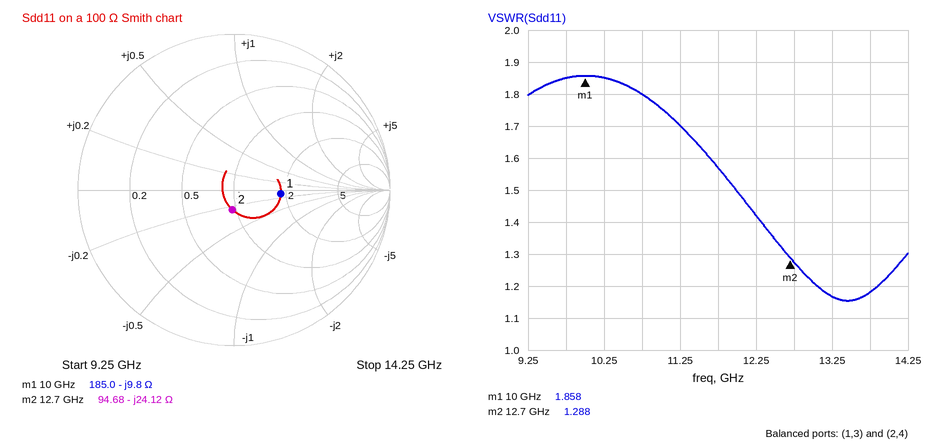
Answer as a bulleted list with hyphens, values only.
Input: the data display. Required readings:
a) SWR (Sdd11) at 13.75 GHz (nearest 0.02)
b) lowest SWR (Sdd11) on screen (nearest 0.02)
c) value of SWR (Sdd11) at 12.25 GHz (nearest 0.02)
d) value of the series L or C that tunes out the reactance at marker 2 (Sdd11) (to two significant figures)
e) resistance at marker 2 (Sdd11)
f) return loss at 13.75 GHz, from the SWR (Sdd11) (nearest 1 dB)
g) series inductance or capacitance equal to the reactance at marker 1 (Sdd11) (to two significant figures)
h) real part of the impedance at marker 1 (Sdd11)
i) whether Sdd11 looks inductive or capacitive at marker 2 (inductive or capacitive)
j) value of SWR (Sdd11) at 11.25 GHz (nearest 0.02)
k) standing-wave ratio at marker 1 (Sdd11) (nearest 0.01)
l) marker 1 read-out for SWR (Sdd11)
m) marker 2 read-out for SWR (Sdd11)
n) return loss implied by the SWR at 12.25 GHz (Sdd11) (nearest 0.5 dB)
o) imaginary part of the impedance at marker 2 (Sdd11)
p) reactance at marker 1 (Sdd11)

- 1.18
- 1.16
- 1.42
- 300 pH
- 94.68 Ω
- 22 dB
- 1.6 pF
- 185.0 Ω
- capacitive
- 1.70
- 1.86
- 1.858
- 1.288
- 15.0 dB
- -24.12 Ω
- -9.8 Ω
